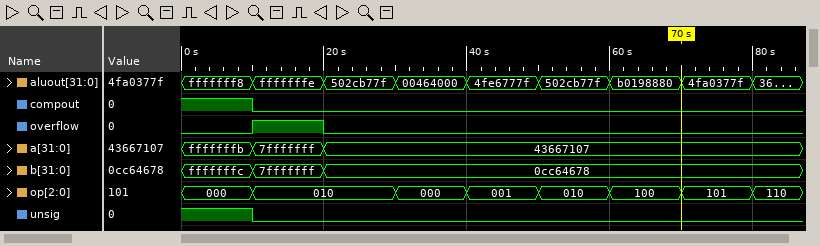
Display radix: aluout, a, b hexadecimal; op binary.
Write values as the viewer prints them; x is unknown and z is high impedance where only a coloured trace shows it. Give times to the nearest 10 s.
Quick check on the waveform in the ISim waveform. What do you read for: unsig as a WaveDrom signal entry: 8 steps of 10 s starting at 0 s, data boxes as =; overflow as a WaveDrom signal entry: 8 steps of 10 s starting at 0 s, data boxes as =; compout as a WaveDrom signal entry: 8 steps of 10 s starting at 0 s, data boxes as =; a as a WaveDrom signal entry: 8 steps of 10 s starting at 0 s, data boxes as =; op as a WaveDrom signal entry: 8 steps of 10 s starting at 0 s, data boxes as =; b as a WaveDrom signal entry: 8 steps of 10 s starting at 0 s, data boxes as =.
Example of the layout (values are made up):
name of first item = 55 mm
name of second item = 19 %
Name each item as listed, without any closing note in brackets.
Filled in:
unsig as a WaveDrom signal entry: 8 steps of 10 s starting at 0 s, data boxes as = = {name: 'unsig', wave: '10......'}
overflow as a WaveDrom signal entry: 8 steps of 10 s starting at 0 s, data boxes as = = {name: 'overflow', wave: '010.....'}
compout as a WaveDrom signal entry: 8 steps of 10 s starting at 0 s, data boxes as = = {name: 'compout', wave: '10......'}
a as a WaveDrom signal entry: 8 steps of 10 s starting at 0 s, data boxes as = = {name: 'a', wave: '===.....', data: 'fffffffb 7fffffff 43667107'}
op as a WaveDrom signal entry: 8 steps of 10 s starting at 0 s, data boxes as = = {name: 'op', wave: '==.=====', data: '000 010 000 001 010 100 101'}
b as a WaveDrom signal entry: 8 steps of 10 s starting at 0 s, data boxes as = = {name: 'b', wave: '===.....', data: 'fffffffc 7fffffff 0cc64678'}
